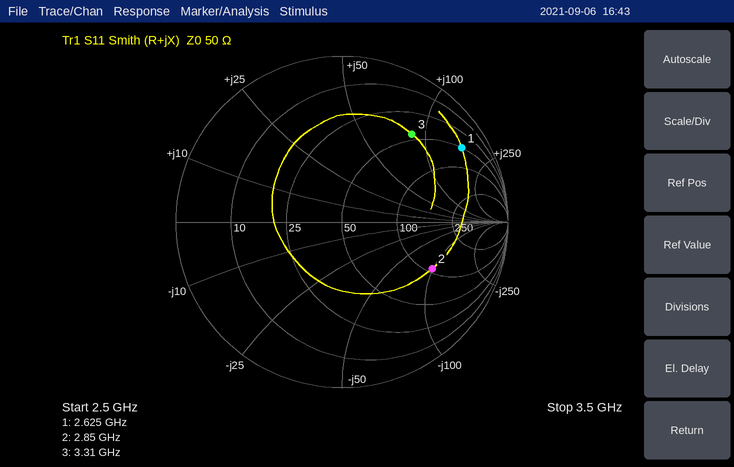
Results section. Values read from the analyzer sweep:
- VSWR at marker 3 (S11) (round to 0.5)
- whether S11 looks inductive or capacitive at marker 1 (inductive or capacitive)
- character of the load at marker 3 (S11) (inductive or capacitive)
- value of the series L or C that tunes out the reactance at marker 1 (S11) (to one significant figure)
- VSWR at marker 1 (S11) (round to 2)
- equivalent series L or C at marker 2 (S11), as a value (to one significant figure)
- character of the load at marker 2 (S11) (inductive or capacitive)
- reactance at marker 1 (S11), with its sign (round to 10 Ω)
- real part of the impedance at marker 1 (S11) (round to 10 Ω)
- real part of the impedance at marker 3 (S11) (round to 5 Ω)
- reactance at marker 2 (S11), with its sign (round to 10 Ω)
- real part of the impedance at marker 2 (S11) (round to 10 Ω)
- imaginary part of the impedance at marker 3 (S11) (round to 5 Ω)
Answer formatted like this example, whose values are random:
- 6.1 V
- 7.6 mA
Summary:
- 5.0
- inductive
- inductive
- 400 fF
- 12
- 600 fF
- capacitive
- +160 Ω
- 50 Ω
- 45 Ω
- -100 Ω
- 110 Ω
- +85 Ω
